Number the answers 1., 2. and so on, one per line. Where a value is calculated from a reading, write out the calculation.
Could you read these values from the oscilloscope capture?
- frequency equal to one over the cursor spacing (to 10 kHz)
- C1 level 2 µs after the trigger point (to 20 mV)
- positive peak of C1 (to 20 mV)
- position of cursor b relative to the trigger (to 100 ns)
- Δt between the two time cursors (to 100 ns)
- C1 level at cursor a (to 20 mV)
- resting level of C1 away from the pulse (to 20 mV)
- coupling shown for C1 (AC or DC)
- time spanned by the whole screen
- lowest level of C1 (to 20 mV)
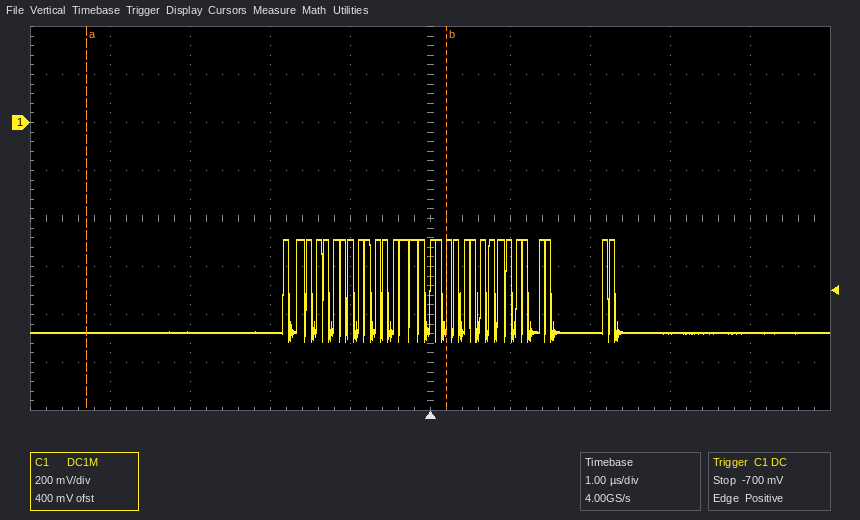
1. 1 / 4.5 µs ≈ 220 kHz
2. -880 mV
3. -480 mV
4. +200 ns
5. 4.5 µs
6. -880 mV
7. -880 mV
8. DC
9. 10 µs
10. -920 mV
